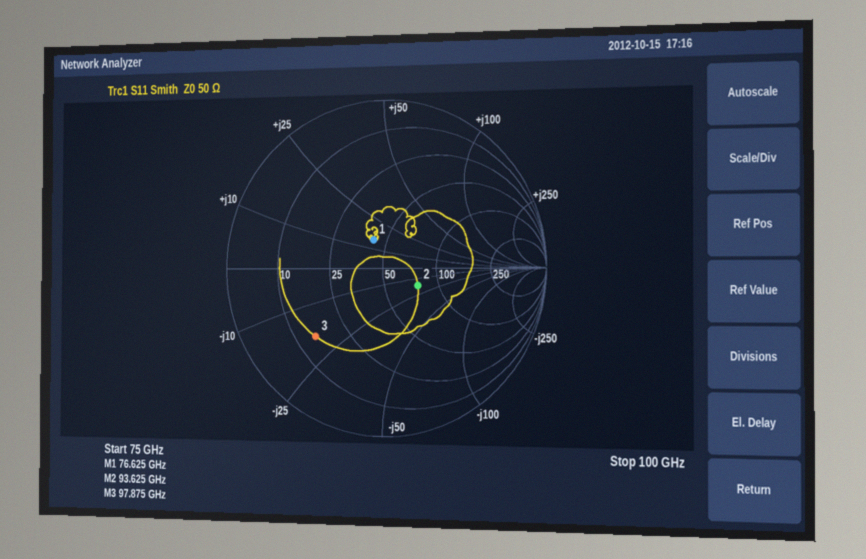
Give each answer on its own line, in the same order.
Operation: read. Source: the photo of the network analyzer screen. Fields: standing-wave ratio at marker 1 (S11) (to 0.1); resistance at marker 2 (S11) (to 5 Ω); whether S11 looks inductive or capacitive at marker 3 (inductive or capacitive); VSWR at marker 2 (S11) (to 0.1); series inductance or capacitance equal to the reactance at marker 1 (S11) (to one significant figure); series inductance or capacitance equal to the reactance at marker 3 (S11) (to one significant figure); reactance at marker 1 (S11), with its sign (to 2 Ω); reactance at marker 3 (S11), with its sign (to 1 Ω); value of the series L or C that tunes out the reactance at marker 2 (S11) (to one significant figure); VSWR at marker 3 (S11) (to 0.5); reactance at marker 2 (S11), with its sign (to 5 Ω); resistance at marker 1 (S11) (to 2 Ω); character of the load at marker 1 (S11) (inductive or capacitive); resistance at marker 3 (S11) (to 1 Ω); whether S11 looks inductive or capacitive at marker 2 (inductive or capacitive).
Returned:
1.4
75 Ω
capacitive
1.6
30 pH
90 fF
+14 Ω
-19 Ω
30 pH
4.0
-15 Ω
42 Ω
inductive
15 Ω
capacitive
